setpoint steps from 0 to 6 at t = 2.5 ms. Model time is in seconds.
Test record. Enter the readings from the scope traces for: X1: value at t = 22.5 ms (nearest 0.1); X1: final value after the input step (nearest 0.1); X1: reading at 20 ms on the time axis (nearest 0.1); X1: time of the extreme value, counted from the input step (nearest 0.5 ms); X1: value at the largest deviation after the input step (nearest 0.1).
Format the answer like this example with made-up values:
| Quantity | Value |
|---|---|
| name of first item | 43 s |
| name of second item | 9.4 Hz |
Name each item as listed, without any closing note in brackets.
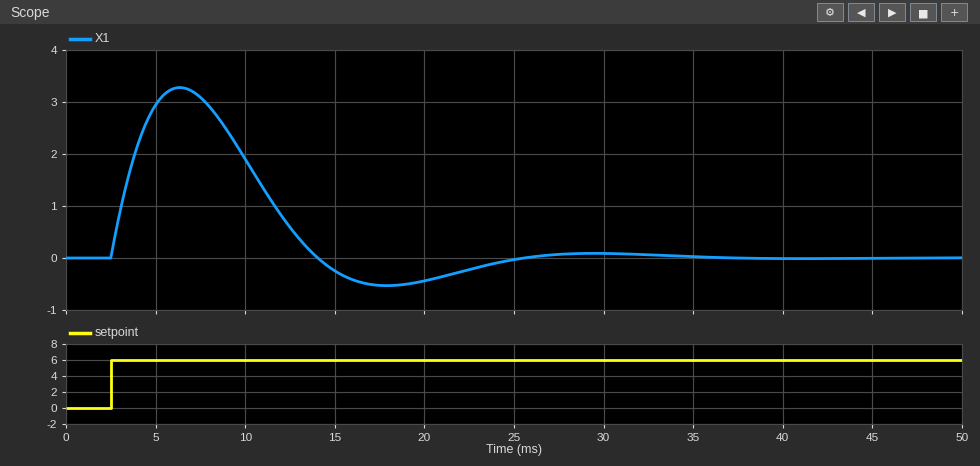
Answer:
| Quantity | Value |
|---|---|
| X1: value at t = 22.5 ms | -0.2 |
| X1: final value after the input step | 0.0 |
| X1: reading at 20 ms on the time axis | -0.4 |
| X1: time of the extreme value, counted from the input step | 4.0 ms |
| X1: value at the largest deviation after the input step | 3.3 |
